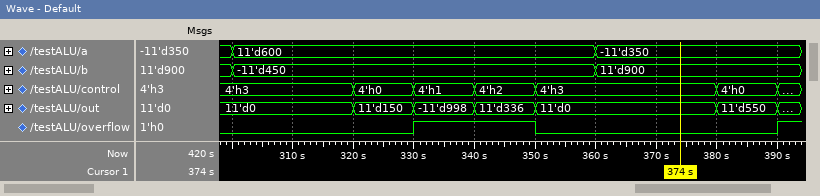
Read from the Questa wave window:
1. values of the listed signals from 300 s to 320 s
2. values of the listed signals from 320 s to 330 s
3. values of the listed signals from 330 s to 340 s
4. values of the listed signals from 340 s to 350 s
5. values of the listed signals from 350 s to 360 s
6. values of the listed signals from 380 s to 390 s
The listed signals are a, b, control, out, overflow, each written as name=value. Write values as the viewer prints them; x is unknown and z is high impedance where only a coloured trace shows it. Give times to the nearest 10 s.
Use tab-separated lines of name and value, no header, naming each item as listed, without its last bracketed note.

values of the listed signals from 300 s to 320 s	a=11'd600, b=-11'd450, control=4'h3, out=11'd0, overflow=0
values of the listed signals from 320 s to 330 s	a=11'd600, b=-11'd450, control=4'h0, out=11'd150, overflow=0
values of the listed signals from 330 s to 340 s	a=11'd600, b=-11'd450, control=4'h1, out=-11'd998, overflow=1
values of the listed signals from 340 s to 350 s	a=11'd600, b=-11'd450, control=4'h2, out=11'd336, overflow=1
values of the listed signals from 350 s to 360 s	a=11'd600, b=-11'd450, control=4'h3, out=11'd0, overflow=0
values of the listed signals from 380 s to 390 s	a=-11'd350, b=11'd900, control=4'h0, out=11'd550, overflow=0
